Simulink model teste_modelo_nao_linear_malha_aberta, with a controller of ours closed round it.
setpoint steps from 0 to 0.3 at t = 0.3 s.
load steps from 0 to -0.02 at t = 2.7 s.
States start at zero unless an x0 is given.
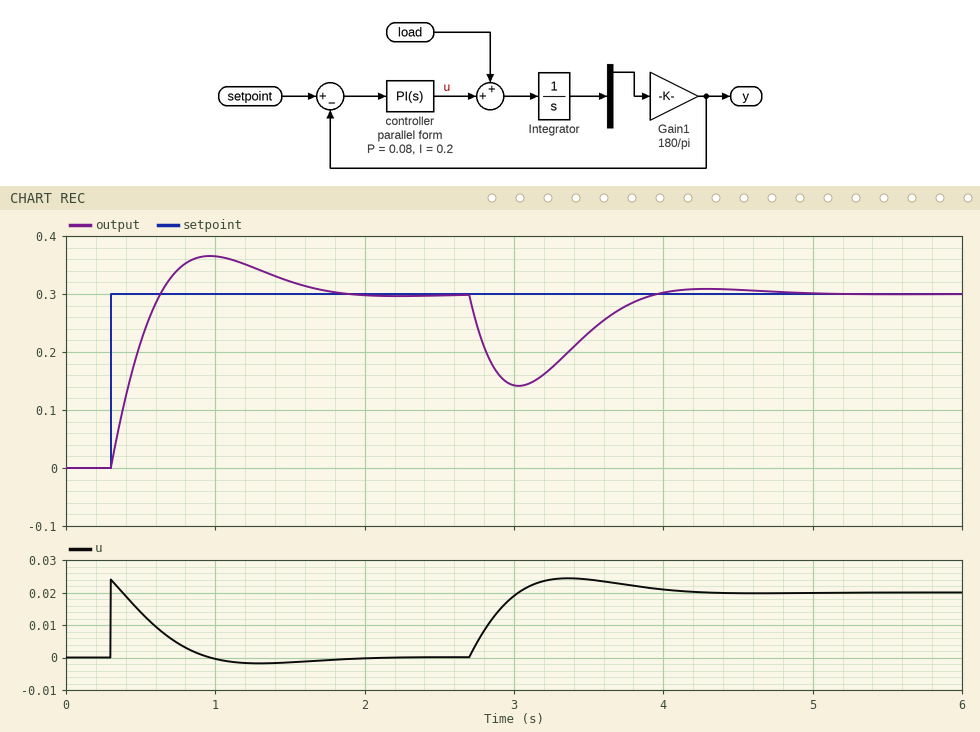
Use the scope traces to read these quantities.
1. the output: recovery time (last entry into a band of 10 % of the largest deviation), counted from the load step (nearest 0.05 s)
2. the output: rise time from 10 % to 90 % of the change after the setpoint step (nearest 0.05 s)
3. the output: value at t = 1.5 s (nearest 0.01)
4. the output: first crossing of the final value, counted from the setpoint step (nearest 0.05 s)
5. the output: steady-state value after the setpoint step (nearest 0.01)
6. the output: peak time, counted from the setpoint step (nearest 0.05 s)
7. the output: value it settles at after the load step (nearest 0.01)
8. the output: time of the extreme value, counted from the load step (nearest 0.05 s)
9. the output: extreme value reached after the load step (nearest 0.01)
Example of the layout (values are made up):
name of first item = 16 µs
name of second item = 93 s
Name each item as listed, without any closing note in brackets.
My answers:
the output: recovery time (last entry into a band of 10 % of the largest deviation), counted from the load step = 1.10 s
the output: rise time from 10 % to 90 % of the change after the setpoint step = 0.25 s
the output: value at t = 1.5 s = 0.32
the output: first crossing of the final value, counted from the setpoint step = 0.35 s
the output: steady-state value after the setpoint step = 0.30
the output: peak time, counted from the setpoint step = 0.65 s
the output: value it settles at after the load step = 0.30
the output: time of the extreme value, counted from the load step = 0.35 s
the output: extreme value reached after the load step = 0.14
